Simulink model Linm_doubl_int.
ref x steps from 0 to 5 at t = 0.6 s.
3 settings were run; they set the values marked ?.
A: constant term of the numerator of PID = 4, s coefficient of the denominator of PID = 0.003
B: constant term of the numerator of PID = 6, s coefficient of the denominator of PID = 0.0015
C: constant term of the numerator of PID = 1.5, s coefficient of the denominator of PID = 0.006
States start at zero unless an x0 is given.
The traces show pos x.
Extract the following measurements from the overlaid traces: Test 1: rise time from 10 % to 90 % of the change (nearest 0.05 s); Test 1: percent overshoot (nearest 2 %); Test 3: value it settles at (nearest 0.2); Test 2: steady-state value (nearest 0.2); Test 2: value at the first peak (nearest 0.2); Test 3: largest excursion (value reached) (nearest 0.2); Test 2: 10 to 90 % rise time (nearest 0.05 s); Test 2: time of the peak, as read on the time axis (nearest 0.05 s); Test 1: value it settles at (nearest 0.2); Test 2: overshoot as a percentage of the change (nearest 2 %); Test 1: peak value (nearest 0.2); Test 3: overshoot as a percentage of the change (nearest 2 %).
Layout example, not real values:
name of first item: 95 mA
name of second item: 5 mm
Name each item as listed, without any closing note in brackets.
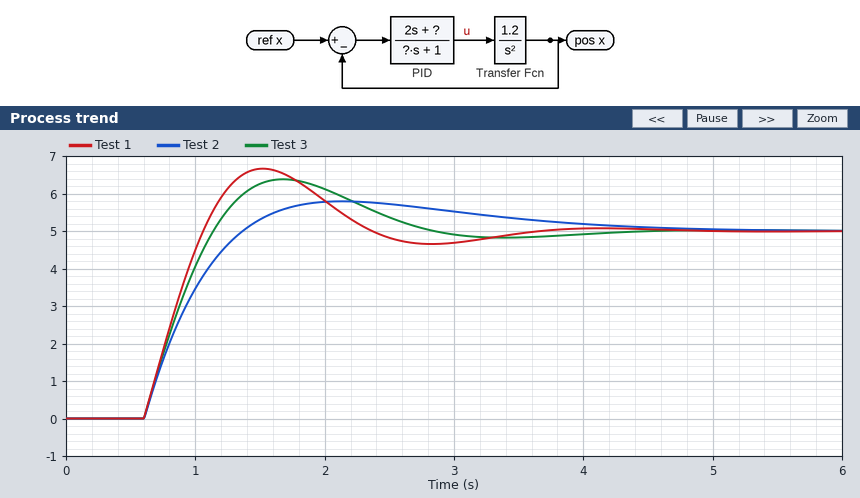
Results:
Test 1: rise time from 10 % to 90 % of the change: 0.35 s
Test 1: percent overshoot: 34 %
Test 3: value it settles at: 5.0
Test 2: steady-state value: 5.0
Test 2: value at the first peak: 5.8
Test 3: largest excursion (value reached): 6.4
Test 2: 10 to 90 % rise time: 0.55 s
Test 2: time of the peak, as read on the time axis: 2.15 s
Test 1: value it settles at: 5.0
Test 2: overshoot as a percentage of the change: 16 %
Test 1: peak value: 6.6
Test 3: overshoot as a percentage of the change: 28 %
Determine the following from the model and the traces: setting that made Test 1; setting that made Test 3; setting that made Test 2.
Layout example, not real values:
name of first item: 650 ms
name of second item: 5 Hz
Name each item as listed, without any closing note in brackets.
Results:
setting that made Test 1: B
setting that made Test 3: A
setting that made Test 2: C
